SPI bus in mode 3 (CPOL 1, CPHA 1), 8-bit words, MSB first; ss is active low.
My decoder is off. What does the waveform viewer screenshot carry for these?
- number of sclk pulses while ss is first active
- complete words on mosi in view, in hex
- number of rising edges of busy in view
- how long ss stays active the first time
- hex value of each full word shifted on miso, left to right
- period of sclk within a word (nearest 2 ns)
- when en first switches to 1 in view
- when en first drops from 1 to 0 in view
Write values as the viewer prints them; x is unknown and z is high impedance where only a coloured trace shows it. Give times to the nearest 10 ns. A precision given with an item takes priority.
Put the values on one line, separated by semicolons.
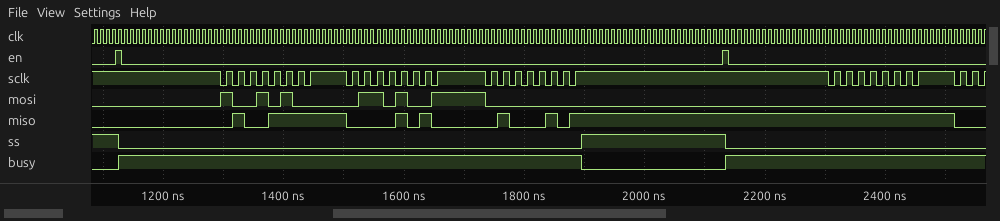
24; 94, 69, 00, 00; 2; 770 ns; 4F, 0A, 45, FF; 20 ns; 1120 ns; 1130 ns
